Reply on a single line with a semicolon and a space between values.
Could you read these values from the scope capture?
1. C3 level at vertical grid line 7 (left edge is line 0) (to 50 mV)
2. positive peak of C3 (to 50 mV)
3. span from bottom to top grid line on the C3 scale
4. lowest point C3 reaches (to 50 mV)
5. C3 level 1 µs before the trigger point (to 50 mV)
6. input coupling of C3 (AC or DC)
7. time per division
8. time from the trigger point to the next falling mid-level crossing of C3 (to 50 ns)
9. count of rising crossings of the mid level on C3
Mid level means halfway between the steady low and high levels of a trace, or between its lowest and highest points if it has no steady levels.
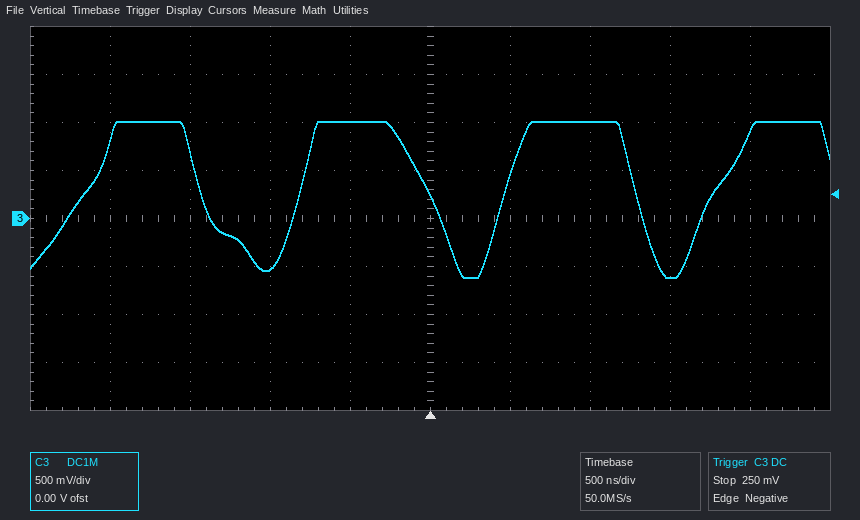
1.00 V; 1.00 V; 4 V; -600 mV; -500 mV; DC; 500 ns; 1.30 µs; 4
